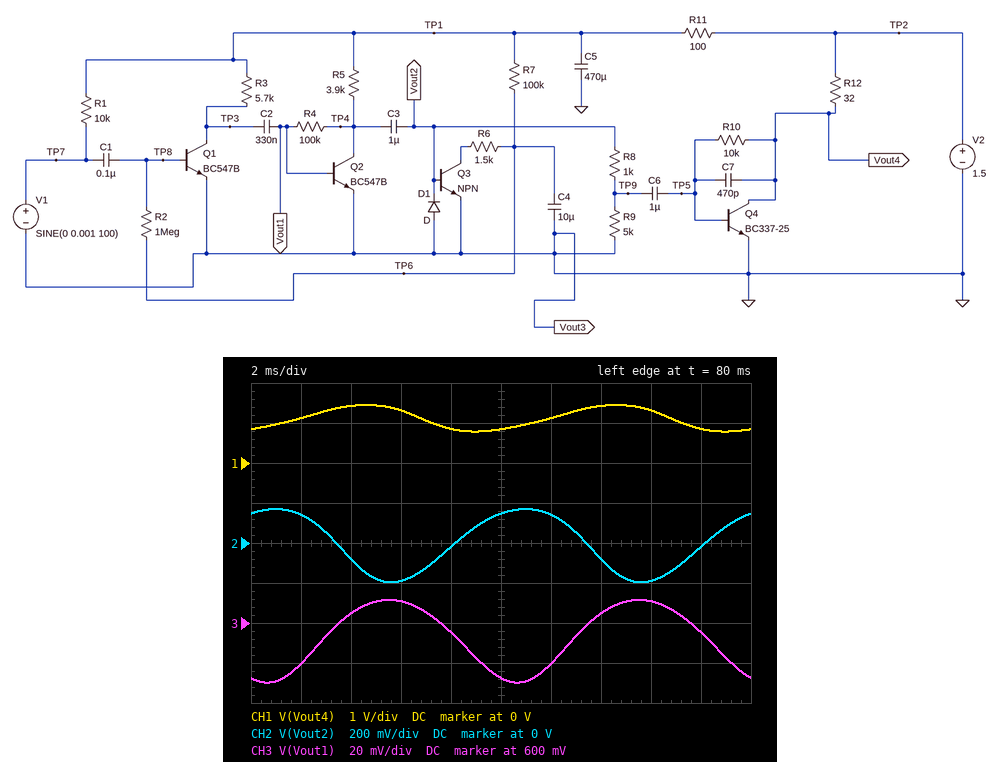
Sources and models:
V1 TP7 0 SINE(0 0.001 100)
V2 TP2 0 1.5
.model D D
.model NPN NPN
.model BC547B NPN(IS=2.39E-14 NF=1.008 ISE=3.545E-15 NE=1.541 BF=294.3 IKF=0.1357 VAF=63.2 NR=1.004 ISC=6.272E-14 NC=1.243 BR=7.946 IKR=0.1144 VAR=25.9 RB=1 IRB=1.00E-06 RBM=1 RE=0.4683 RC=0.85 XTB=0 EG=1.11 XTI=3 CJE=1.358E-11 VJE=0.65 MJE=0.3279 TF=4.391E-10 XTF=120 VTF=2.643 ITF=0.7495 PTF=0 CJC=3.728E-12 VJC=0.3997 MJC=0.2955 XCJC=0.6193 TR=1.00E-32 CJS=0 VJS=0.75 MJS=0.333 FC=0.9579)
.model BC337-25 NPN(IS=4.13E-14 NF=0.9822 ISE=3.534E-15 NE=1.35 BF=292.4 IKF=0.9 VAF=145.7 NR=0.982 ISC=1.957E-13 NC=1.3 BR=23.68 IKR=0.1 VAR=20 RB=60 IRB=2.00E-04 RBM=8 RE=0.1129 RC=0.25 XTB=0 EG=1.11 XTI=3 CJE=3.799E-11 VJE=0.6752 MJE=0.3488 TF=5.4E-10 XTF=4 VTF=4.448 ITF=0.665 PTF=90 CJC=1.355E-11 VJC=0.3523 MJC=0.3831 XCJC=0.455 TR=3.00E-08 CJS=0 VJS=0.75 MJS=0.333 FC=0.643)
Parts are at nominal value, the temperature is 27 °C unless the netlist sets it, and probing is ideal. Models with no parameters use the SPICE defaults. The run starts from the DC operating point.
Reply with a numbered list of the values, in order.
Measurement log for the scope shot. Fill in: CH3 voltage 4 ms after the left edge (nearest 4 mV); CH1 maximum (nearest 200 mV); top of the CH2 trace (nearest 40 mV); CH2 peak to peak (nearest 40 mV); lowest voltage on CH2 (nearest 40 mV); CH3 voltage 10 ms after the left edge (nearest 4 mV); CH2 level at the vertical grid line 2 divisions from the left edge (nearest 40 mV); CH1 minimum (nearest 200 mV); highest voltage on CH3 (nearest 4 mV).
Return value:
1. 604 mV
2. 1.4 V
3. 160 mV
4. 360 mV
5. -200 mV
6. 572 mV
7. -80 mV
8. 800 mV
9. 612 mV
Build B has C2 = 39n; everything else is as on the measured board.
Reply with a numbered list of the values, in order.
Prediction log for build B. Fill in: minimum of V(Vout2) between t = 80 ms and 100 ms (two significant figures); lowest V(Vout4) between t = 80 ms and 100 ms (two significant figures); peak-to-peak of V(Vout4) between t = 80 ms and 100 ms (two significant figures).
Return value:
1. -44 mV
2. 1.0 V
3. 190 mV
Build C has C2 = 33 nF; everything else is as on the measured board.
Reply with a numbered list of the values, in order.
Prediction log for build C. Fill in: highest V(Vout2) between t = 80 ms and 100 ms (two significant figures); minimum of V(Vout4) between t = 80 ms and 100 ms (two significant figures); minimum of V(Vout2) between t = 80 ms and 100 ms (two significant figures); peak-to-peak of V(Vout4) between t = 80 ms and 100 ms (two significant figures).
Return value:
1. 44 mV
2. 1.0 V
3. -37 mV
4. 160 mV
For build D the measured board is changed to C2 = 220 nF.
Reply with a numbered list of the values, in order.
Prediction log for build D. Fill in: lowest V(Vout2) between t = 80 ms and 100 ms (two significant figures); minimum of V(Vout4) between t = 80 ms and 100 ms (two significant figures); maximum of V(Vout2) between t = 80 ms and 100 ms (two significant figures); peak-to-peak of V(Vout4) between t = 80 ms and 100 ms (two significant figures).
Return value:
1. -180 mV
2. 810 mV
3. 160 mV
4. 630 mV
